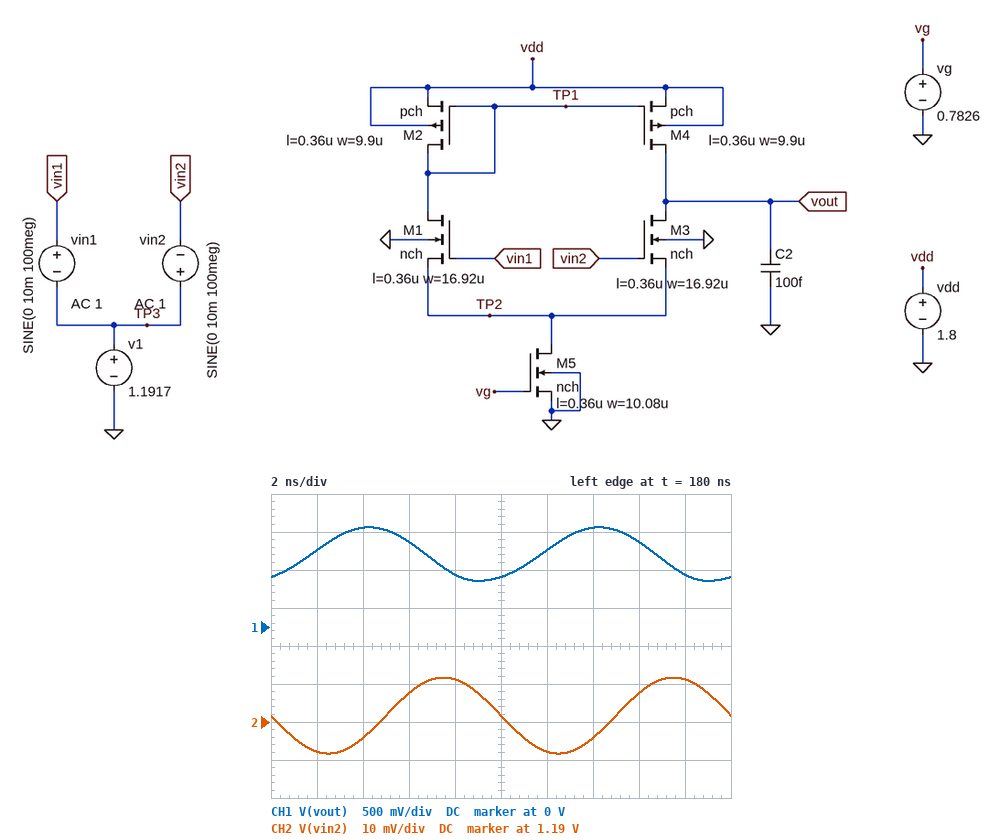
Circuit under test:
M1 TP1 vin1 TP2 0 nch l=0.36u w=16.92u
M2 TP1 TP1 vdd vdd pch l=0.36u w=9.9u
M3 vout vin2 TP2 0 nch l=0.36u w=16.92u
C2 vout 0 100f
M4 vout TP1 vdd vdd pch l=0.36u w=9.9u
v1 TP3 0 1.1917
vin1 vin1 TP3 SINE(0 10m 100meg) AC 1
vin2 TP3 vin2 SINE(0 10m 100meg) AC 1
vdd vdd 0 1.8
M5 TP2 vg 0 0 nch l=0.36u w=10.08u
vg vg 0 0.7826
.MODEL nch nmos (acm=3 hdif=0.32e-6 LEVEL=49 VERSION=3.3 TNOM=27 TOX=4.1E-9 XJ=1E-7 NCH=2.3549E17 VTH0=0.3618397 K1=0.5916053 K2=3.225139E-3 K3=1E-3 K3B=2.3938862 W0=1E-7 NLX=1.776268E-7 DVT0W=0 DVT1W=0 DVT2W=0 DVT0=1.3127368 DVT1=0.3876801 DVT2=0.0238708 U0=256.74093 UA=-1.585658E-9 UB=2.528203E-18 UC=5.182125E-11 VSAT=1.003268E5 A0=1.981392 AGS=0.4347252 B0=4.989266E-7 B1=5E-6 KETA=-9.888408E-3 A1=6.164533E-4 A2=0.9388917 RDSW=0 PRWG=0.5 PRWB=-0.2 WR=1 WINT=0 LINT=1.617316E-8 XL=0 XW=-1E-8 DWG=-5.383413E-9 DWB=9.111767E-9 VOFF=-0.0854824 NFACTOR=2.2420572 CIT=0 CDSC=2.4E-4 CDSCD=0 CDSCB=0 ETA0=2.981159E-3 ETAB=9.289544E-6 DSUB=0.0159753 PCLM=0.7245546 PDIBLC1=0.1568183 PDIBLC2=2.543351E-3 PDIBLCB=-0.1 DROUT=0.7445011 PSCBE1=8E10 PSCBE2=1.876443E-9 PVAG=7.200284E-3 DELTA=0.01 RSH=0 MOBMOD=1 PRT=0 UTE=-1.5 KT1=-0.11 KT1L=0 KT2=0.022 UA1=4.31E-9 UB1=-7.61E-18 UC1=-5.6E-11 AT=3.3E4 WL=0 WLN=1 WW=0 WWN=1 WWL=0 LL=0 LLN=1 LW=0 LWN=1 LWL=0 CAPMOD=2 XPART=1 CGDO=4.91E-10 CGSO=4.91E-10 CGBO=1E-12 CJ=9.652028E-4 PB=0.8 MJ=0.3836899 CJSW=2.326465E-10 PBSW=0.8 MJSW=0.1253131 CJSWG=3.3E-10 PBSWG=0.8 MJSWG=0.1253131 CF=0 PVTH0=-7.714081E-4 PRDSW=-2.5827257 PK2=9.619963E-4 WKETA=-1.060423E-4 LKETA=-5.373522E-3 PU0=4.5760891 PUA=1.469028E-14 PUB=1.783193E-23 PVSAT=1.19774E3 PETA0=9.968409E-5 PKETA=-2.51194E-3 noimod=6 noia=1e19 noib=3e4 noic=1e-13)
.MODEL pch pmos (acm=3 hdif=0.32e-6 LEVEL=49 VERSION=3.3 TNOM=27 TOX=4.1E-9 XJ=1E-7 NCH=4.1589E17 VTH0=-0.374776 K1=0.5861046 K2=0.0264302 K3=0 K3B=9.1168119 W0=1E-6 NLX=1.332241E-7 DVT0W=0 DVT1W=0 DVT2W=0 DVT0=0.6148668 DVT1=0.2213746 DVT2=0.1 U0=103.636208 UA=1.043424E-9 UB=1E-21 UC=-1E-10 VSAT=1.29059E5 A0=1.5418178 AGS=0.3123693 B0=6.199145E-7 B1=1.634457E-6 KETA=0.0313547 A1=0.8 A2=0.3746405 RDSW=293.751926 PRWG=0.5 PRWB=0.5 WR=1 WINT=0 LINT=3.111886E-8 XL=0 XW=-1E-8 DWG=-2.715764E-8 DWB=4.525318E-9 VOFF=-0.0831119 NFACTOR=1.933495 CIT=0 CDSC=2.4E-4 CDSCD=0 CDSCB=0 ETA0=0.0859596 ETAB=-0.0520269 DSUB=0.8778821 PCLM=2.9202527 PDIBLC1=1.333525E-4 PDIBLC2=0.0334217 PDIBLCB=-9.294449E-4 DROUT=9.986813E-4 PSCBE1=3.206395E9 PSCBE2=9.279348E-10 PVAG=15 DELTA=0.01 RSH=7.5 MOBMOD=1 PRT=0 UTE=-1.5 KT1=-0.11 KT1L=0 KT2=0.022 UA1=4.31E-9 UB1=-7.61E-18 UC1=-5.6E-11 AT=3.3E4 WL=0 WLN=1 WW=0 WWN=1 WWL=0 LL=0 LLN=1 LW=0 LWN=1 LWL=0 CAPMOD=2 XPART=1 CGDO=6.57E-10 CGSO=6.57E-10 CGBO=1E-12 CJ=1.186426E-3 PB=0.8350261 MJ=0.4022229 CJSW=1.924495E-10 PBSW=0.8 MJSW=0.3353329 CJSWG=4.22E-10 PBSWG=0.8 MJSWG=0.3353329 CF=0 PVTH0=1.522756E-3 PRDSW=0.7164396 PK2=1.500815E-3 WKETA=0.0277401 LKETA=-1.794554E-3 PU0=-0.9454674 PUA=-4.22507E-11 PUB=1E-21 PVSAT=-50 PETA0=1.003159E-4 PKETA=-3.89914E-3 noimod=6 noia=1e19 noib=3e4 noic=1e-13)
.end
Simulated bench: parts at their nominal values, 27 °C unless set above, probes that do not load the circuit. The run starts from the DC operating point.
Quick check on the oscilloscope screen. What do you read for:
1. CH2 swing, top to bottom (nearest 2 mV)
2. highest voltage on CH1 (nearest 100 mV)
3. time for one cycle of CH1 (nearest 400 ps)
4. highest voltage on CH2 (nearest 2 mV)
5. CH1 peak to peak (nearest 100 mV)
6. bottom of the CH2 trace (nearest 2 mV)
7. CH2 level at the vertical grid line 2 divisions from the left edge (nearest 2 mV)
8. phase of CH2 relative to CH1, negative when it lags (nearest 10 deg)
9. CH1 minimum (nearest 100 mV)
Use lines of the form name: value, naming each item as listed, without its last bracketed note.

CH2 swing, top to bottom: 20 mV
highest voltage on CH1: 1.3 V
time for one cycle of CH1: 10.0 ns
highest voltage on CH2: 1.202 V
CH1 peak to peak: 700 mV
bottom of the CH2 trace: 1.182 V
CH2 level at the vertical grid line 2 divisions from the left edge: 1.186 V
phase of CH2 relative to CH1, negative when it lags: -120 deg
CH1 minimum: 600 mV
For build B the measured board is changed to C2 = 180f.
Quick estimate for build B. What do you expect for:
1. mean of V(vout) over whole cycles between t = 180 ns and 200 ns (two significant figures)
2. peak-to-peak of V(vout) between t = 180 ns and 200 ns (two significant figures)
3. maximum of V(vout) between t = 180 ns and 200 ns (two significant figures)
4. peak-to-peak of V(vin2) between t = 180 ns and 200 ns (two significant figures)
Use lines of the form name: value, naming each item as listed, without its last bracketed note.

mean of V(vout) over whole cycles between t = 180 ns and 200 ns: 940 mV
peak-to-peak of V(vout) between t = 180 ns and 200 ns: 500 mV
maximum of V(vout) between t = 180 ns and 200 ns: 1.2 V
peak-to-peak of V(vin2) between t = 180 ns and 200 ns: 20 mV
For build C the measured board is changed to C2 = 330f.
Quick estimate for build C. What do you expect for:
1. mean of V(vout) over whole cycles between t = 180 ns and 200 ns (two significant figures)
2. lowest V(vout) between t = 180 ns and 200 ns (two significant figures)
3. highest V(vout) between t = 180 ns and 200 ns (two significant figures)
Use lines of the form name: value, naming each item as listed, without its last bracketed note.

mean of V(vout) over whole cycles between t = 180 ns and 200 ns: 930 mV
lowest V(vout) between t = 180 ns and 200 ns: 770 mV
highest V(vout) between t = 180 ns and 200 ns: 1.1 V
